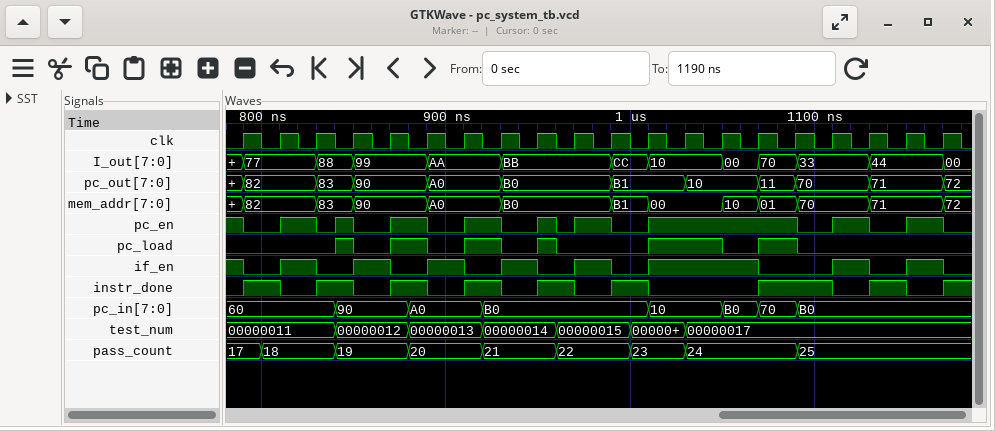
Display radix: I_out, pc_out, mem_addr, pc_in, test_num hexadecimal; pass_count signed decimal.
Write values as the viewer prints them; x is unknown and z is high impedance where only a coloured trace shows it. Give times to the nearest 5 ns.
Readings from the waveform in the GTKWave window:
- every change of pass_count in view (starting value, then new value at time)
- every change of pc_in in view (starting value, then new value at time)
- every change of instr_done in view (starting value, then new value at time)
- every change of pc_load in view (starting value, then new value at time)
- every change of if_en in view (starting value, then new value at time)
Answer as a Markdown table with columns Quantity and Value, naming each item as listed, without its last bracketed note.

| Quantity | Value |
|---|---|
| every change of pass_count in view | 17, 18 at 800 ns, 19 at 840 ns, 20 at 880 ns, 21 at 920 ns, 22 at 960 ns, 23 at 1000 ns, 24 at 1030 ns, 25 at 1090 ns |
| every change of pc_in in view | 60, 90 at 840 ns, A0 at 880 ns, B0 at 920 ns, 10 at 1010 ns, B0 at 1050 ns, 70 at 1070 ns, B0 at 1090 ns |
| every change of instr_done in view | 0, 1 at 790 ns, 0 at 810 ns, 1 at 830 ns, 0 at 850 ns, 1 at 870 ns, 0 at 890 ns, 1 at 910 ns, 0 at 930 ns, 1 at 950 ns, 0 at 970 ns, 1 at 990 ns, 0 at 1010 ns, 1 at 1070 ns, 0 at 1110 ns, 1 at 1130 ns, 0 at 1150 ns, 1 at 1170 ns |
| every change of pc_load in view | 0, 1 at 840 ns, 0 at 850 ns, 1 at 870 ns, 0 at 890 ns, 1 at 910 ns, 0 at 930 ns, 1 at 950 ns, 0 at 960 ns, 1 at 1010 ns, 0 at 1050 ns, 1 at 1070 ns, 0 at 1090 ns |
| every change of if_en in view | 1, 0 at 790 ns, 1 at 810 ns, 0 at 830 ns, 1 at 850 ns, 0 at 870 ns, 1 at 890 ns, 0 at 910 ns, 1 at 930 ns, 0 at 950 ns, 1 at 970 ns, 0 at 990 ns, 1 at 1010 ns, 0 at 1070 ns, 1 at 1110 ns, 0 at 1130 ns, 1 at 1150 ns, 0 at 1170 ns |
